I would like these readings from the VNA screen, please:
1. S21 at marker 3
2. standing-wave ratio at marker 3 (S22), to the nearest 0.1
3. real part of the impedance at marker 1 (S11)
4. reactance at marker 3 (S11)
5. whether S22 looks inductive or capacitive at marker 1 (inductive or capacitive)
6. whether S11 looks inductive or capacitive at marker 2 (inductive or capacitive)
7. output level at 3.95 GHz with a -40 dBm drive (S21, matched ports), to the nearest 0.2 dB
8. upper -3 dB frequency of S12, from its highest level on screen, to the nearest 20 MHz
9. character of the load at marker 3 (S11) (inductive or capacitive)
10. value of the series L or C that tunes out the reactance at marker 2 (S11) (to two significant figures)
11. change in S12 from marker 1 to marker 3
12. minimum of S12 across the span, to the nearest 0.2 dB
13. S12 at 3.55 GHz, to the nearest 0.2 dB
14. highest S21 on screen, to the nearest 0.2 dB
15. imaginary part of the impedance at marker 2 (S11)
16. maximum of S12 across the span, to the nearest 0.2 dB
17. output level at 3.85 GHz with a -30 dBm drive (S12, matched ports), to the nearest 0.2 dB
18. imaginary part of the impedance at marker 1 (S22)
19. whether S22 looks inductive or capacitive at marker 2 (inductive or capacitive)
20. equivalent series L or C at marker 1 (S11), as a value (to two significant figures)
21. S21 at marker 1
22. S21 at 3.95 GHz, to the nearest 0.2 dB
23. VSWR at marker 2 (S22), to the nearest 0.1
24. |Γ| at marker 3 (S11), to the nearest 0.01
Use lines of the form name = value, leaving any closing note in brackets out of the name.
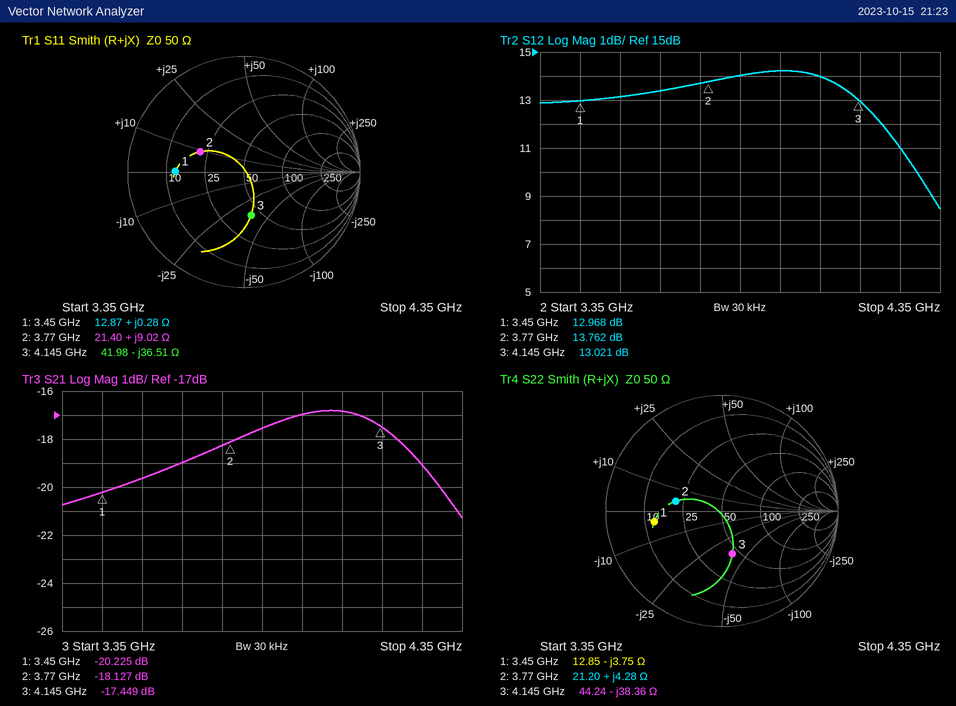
S21 at marker 3 = -17.449 dB
standing-wave ratio at marker 3 (S22), to the nearest 0.1 = 2.2
real part of the impedance at marker 1 = 12.87 Ω
reactance at marker 3 = -36.51 Ω
whether S22 looks inductive or capacitive at marker 1 = capacitive
whether S11 looks inductive or capacitive at marker 2 = inductive
output level at 3.95 GHz with a -40 dBm drive (S21, matched ports), to the nearest 0.2 dB = -57.0 dBm
upper -3 dB frequency of S12, from its highest level on screen, to the nearest 20 MHz = 4.24 GHz
character of the load at marker 3 (S11) = capacitive
value of the series L or C that tunes out the reactance at marker 2 (S11) = 4.7 pF
change in S12 from marker 1 to marker 3 = 0.053 dB
minimum of S12 across the span, to the nearest 0.2 dB = 8.4 dB
S12 at 3.55 GHz, to the nearest 0.2 dB = 13.2 dB
highest S21 on screen, to the nearest 0.2 dB = -16.8 dB
imaginary part of the impedance at marker 2 = +9.02 Ω
maximum of S12 across the span, to the nearest 0.2 dB = 14.2 dB
output level at 3.85 GHz with a -30 dBm drive (S12, matched ports), to the nearest 0.2 dB = -16.0 dBm
imaginary part of the impedance at marker 1 = -3.75 Ω
whether S22 looks inductive or capacitive at marker 2 = inductive
equivalent series L or C at marker 1 (S11), as a value = 13 pH
S21 at marker 1 = -20.225 dB
S21 at 3.95 GHz, to the nearest 0.2 dB = -17.0 dB
VSWR at marker 2 (S22), to the nearest 0.1 = 2.4
|Γ| at marker 3 (S11), to the nearest 0.01 = 0.38
